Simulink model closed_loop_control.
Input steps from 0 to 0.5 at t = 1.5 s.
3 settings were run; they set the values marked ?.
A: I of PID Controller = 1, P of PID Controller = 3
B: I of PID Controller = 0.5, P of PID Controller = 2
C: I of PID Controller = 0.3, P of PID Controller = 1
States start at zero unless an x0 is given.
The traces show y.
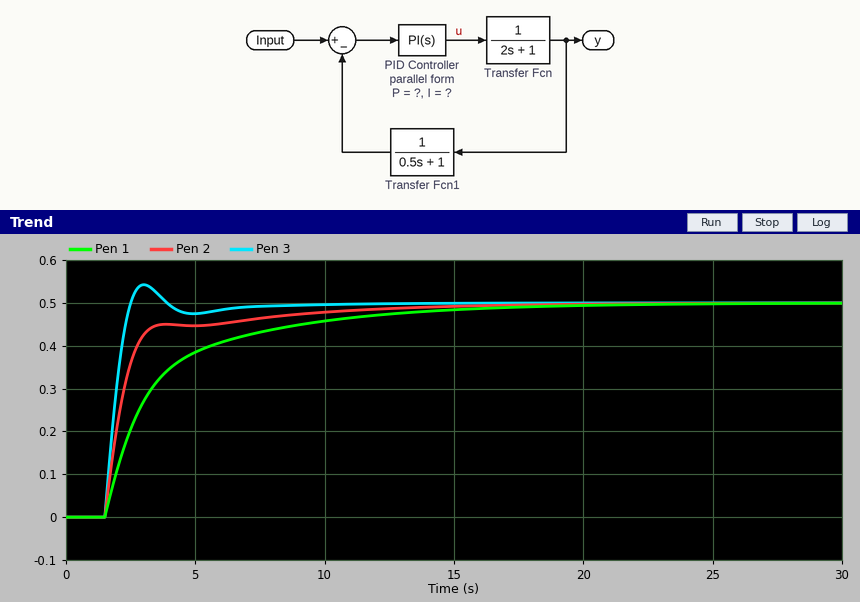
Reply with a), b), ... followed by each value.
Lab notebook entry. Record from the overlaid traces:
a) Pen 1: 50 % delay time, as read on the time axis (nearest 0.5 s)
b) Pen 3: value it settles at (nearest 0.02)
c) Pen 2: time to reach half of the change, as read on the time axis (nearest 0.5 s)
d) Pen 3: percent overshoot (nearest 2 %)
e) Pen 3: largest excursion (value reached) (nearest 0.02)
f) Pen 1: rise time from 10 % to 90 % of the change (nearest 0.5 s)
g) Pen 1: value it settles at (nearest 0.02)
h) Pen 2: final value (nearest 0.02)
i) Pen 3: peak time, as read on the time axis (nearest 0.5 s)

a) 3.0 s
b) 0.50
c) 2.0 s
d) 8 %
e) 0.54
f) 7.5 s
g) 0.50
h) 0.50
i) 3.0 s
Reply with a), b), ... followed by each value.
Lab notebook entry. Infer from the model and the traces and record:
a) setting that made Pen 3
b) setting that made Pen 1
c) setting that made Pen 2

a) A
b) C
c) B
